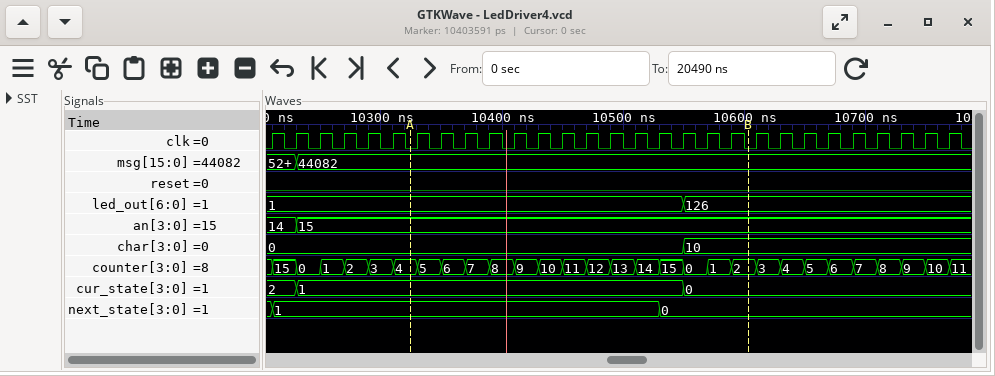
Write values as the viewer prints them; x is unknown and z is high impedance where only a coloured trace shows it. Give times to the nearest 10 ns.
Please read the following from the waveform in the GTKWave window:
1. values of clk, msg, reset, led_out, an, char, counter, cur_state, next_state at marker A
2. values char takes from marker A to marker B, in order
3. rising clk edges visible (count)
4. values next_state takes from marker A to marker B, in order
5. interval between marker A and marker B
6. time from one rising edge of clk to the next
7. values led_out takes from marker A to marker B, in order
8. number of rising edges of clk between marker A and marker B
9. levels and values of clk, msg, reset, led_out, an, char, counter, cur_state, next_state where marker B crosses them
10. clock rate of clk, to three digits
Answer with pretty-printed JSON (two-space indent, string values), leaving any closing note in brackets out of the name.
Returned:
{
  "values of clk, msg, reset, led_out, an, char, counter, cur_state, next_state at marker A": "clk=0, msg=44082, reset=0, led_out=1, an=15, char=0, counter=4, cur_state=1, next_state=1",
  "values char takes from marker A to marker B, in order": "0, 10",
  "rising clk edges visible": "29",
  "values next_state takes from marker A to marker B, in order": "1, 0",
  "interval between marker A and marker B": "280 ns",
  "time from one rising edge of clk to the next": "20 ns",
  "values led_out takes from marker A to marker B, in order": "1, 126",
  "number of rising edges of clk between marker A and marker B": "14",
  "levels and values of clk, msg, reset, led_out, an, char, counter, cur_state, next_state where marker B crosses them": "clk=0, msg=44082, reset=0, led_out=126, an=15, char=10, counter=2, cur_state=0, next_state=0",
  "clock rate of clk, to three digits": "50.0 MHz"
}
